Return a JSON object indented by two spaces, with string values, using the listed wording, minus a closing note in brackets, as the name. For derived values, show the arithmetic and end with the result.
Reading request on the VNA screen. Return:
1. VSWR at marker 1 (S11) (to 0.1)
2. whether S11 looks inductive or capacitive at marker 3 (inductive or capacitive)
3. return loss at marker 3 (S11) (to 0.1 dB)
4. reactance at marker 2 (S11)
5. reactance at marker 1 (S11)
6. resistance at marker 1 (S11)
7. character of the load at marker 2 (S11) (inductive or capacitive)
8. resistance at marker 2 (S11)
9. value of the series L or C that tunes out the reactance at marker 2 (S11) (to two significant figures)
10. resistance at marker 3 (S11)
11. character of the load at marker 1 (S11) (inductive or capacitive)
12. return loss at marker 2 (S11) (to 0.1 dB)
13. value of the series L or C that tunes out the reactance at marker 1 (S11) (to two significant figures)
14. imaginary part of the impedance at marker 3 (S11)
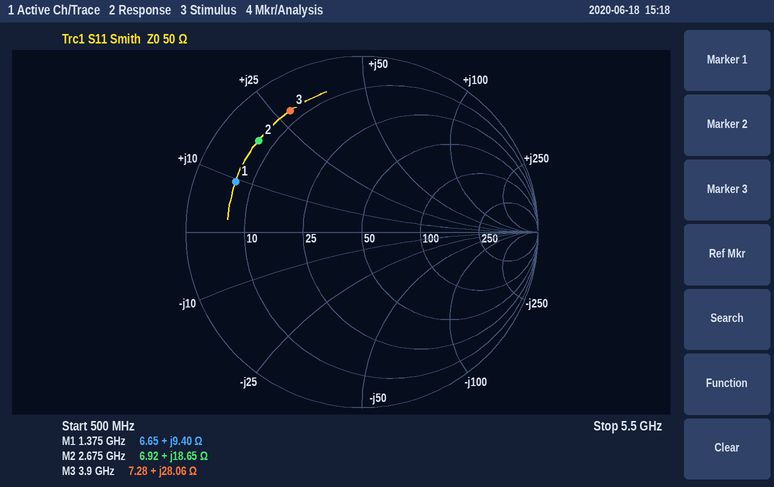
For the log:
{
  "VSWR at marker 1 (S11)": "7.8",
  "whether S11 looks inductive or capacitive at marker 3": "inductive",
  "return loss at marker 3 (S11)": "1.9 dB",
  "reactance at marker 2": "+18.65 Ω",
  "reactance at marker 1": "+9.40 Ω",
  "resistance at marker 1": "6.65 Ω",
  "character of the load at marker 2 (S11)": "inductive",
  "resistance at marker 2": "6.92 Ω",
  "value of the series L or C that tunes out the reactance at marker 2 (S11)": "C = 1/(2π × 2.675 GHz × 18.65 Ω) ≈ 3.2 pF",
  "resistance at marker 3": "7.28 Ω",
  "character of the load at marker 1 (S11)": "inductive",
  "return loss at marker 2 (S11)": "2.1 dB",
  "value of the series L or C that tunes out the reactance at marker 1 (S11)": "C = 1/(2π × 1.375 GHz × 9.4 Ω) ≈ 12 pF",
  "imaginary part of the impedance at marker 3": "+28.06 Ω"
}
